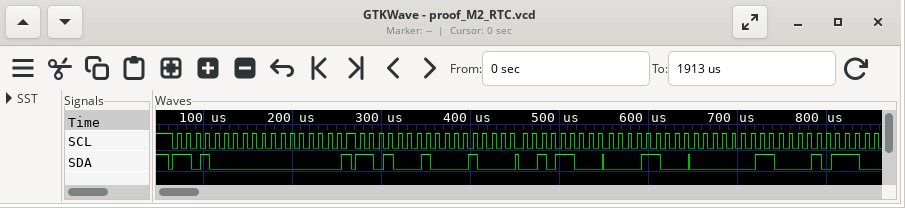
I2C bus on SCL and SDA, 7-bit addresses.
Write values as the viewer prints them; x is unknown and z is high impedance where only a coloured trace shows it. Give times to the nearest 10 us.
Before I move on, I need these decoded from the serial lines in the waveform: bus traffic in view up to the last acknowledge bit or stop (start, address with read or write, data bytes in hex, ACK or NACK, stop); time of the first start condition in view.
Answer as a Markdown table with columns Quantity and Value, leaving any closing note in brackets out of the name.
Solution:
| Quantity | Value |
|---|---|
| bus traffic in view up to the last acknowledge bit or stop | start, address 68 write ACK, 00 ACK, repeated start, address 68 read ACK, 10 ACK, 58 ACK, 18 ACK, 03 ACK, 17 ACK |
| time of the first start condition in view | 60 us |
